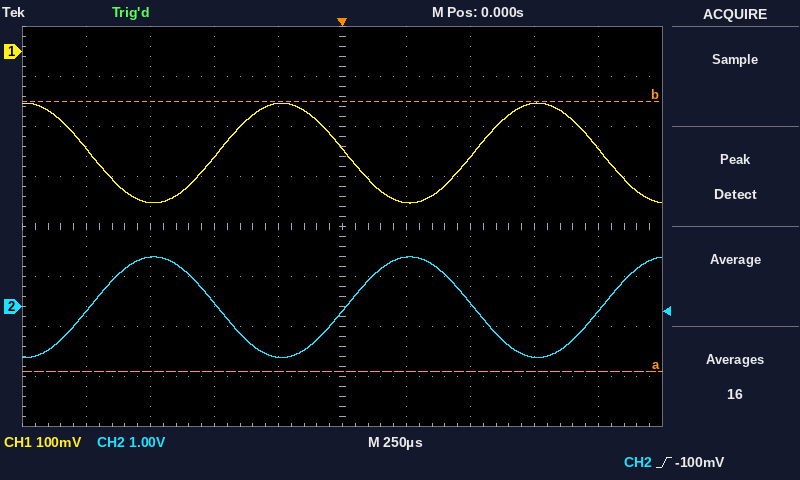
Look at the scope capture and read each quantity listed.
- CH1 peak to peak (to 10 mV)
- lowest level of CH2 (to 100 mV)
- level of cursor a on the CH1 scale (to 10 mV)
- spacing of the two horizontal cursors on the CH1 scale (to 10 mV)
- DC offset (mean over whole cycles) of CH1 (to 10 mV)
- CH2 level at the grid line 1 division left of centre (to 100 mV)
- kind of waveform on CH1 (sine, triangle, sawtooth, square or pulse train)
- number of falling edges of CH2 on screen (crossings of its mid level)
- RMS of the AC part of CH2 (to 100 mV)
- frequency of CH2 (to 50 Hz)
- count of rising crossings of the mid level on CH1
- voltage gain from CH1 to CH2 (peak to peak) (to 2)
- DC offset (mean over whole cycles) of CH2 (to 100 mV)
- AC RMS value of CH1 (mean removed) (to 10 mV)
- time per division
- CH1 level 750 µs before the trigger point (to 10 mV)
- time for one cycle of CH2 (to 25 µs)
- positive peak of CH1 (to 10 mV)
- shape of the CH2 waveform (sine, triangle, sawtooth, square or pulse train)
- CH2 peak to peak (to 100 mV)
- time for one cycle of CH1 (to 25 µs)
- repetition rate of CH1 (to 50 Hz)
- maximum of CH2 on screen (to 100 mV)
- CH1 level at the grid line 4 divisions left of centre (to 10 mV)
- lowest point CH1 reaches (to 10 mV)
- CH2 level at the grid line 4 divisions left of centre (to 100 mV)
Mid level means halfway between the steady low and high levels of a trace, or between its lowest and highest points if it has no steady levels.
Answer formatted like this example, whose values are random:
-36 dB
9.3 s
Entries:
200 mV
-1.0 V
-640 mV
540 mV
-200 mV
-1.0 V
sine
2
700 mV
1.00 kHz
2
10
0.0 V
70 mV
250 µs
-300 mV
1.000 ms
-100 mV
sine
2.0 V
1.000 ms
1.00 kHz
1.0 V
-190 mV
-300 mV
-100 mV
